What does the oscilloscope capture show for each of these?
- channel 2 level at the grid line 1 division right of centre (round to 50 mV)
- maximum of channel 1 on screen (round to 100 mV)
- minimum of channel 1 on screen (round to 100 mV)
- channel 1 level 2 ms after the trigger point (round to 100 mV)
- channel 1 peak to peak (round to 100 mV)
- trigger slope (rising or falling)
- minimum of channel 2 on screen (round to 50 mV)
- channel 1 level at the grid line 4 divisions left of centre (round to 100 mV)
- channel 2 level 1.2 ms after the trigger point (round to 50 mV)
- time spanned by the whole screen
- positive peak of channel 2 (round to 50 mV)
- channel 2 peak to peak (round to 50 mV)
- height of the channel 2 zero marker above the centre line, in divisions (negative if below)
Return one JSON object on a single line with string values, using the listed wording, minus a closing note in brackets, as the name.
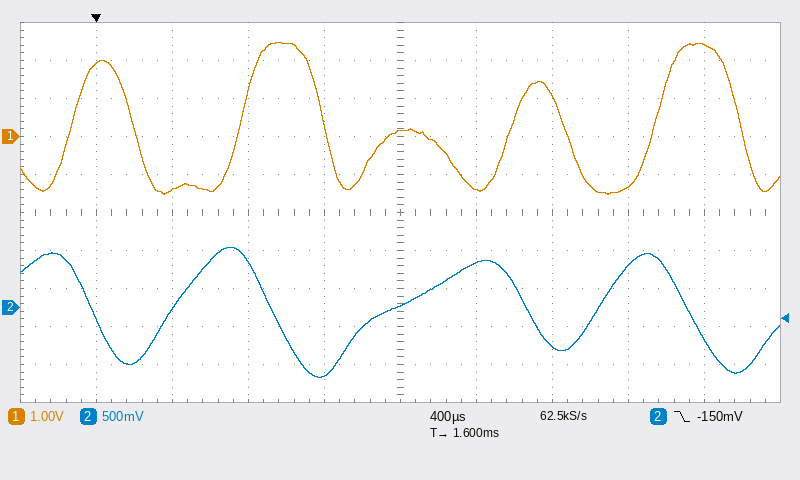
{"channel 2 level at the grid line 1 division right of centre": "600 mV", "maximum of channel 1 on screen": "2.5 V", "minimum of channel 1 on screen": "-1.5 V", "channel 1 level 2 ms after the trigger point": "-1.4 V", "channel 1 peak to peak": "4.0 V", "trigger slope": "falling", "minimum of channel 2 on screen": "-900 mV", "channel 1 level at the grid line 4 divisions left of centre": "1.9 V", "channel 2 level 1.2 ms after the trigger point": "-900 mV", "time spanned by the whole screen": "4 ms", "positive peak of channel 2": "800 mV", "channel 2 peak to peak": "1.70 V", "height of the channel 2 zero marker above the centre line, in divisions": "-2.5 div"}
